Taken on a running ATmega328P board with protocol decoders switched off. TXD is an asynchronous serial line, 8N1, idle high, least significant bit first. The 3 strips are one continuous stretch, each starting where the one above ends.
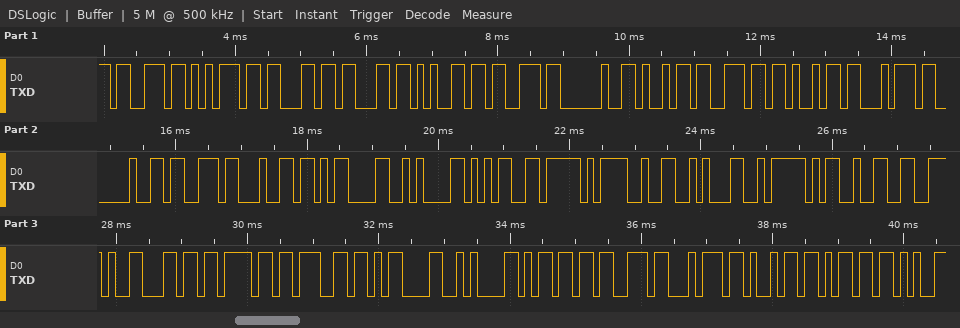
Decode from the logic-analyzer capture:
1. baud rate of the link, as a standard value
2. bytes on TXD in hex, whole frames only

9600 baud
73 75 63 63 65 73 20 69 6E 69 74 20 73 64 0D 0A 35 5F 32 31 5F 32 2E 6C 6F 67 0D 0A 6D 73 74 69 6D
